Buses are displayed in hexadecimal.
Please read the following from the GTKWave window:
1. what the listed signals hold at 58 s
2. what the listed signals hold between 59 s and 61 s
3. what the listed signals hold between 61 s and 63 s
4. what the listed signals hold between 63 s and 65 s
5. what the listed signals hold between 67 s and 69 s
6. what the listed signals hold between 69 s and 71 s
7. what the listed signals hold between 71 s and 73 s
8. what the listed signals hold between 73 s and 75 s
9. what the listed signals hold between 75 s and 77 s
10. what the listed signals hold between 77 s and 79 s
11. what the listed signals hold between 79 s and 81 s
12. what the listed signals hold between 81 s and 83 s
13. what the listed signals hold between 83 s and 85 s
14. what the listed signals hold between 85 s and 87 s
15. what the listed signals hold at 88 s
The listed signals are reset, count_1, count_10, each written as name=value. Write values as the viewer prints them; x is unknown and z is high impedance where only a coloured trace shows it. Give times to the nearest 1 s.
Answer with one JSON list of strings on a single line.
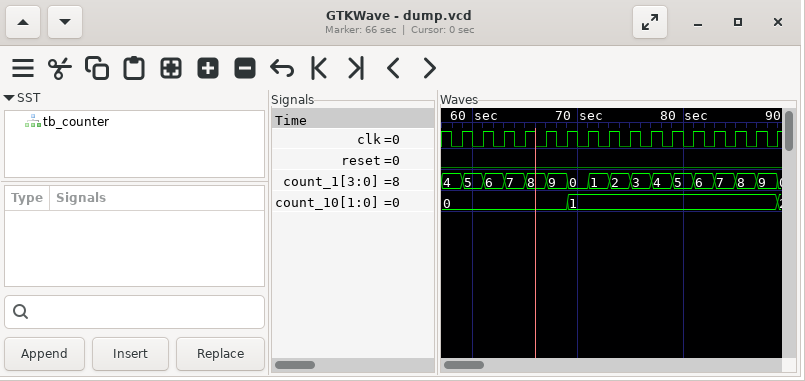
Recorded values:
["reset=0, count_1=4, count_10=0", "reset=0, count_1=5, count_10=0", "reset=0, count_1=6, count_10=0", "reset=0, count_1=7, count_10=0", "reset=0, count_1=9, count_10=0", "reset=0, count_1=0, count_10=1", "reset=0, count_1=1, count_10=1", "reset=0, count_1=2, count_10=1", "reset=0, count_1=3, count_10=1", "reset=0, count_1=4, count_10=1", "reset=0, count_1=5, count_10=1", "reset=0, count_1=6, count_10=1", "reset=0, count_1=7, count_10=1", "reset=0, count_1=8, count_10=1", "reset=0, count_1=9, count_10=1"]
